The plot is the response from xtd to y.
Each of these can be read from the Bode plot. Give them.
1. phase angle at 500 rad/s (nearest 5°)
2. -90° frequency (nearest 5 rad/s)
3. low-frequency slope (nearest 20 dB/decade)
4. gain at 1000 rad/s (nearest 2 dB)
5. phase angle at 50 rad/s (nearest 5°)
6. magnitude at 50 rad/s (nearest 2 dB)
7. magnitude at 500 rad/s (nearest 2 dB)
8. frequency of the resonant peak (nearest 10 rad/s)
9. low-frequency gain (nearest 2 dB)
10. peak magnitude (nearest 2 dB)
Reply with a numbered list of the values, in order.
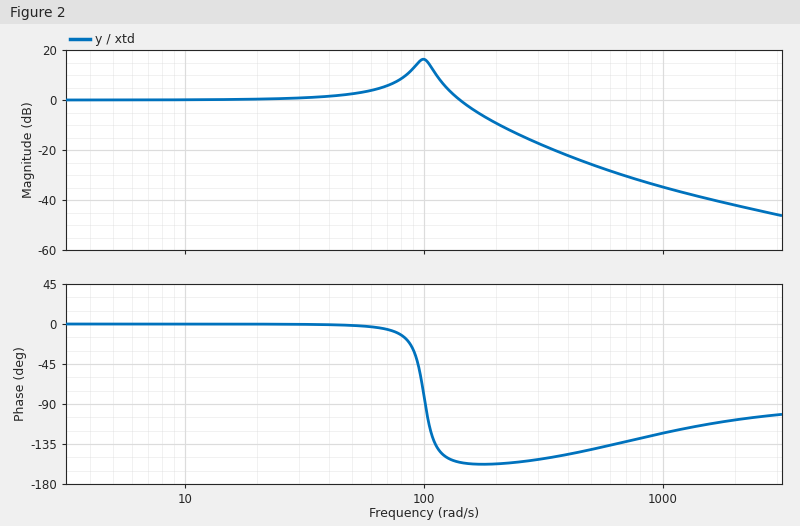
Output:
1. -140°
2. 100 rad/s
3. 0 dB/decade
4. -34 dB
5. 0°
6. 2 dB
7. -26 dB
8. 100 rad/s
9. 0 dB
10. 16 dB
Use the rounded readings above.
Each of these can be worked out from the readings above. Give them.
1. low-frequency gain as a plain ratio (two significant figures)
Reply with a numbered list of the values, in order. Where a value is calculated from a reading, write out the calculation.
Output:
1. 10^(0 / 20) = 1.0
